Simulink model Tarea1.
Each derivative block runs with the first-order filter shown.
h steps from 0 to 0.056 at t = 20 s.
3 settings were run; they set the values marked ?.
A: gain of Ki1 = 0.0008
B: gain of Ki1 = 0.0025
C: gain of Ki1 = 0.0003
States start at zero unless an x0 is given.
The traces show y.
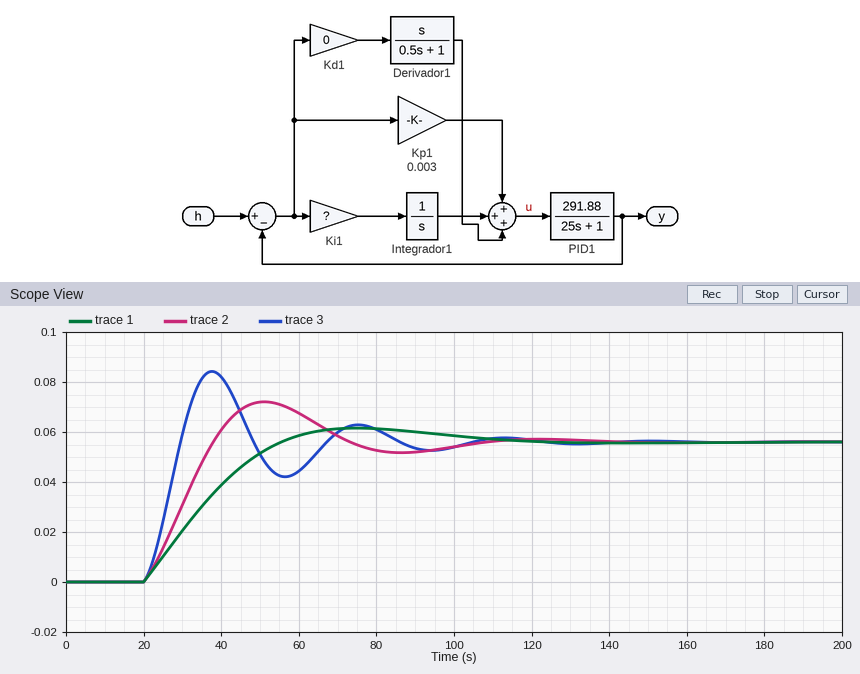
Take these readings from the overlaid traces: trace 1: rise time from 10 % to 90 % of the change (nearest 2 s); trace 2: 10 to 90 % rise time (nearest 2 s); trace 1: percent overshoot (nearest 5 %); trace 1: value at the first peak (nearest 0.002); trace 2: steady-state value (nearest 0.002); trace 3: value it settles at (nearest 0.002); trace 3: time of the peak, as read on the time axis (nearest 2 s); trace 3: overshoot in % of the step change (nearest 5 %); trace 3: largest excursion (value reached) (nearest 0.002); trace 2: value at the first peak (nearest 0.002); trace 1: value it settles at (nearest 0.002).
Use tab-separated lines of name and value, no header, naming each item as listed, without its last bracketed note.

trace 1: rise time from 10 % to 90 % of the change	26 s
trace 2: 10 to 90 % rise time	14 s
trace 1: percent overshoot	10 %
trace 1: value at the first peak	0.062
trace 2: steady-state value	0.056
trace 3: value it settles at	0.056
trace 3: time of the peak, as read on the time axis	38 s
trace 3: overshoot in % of the step change	50 %
trace 3: largest excursion (value reached)	0.084
trace 2: value at the first peak	0.072
trace 1: value it settles at	0.056
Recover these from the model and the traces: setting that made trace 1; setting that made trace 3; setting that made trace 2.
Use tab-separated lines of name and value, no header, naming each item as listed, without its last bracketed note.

setting that made trace 1	C
setting that made trace 3	B
setting that made trace 2	A
